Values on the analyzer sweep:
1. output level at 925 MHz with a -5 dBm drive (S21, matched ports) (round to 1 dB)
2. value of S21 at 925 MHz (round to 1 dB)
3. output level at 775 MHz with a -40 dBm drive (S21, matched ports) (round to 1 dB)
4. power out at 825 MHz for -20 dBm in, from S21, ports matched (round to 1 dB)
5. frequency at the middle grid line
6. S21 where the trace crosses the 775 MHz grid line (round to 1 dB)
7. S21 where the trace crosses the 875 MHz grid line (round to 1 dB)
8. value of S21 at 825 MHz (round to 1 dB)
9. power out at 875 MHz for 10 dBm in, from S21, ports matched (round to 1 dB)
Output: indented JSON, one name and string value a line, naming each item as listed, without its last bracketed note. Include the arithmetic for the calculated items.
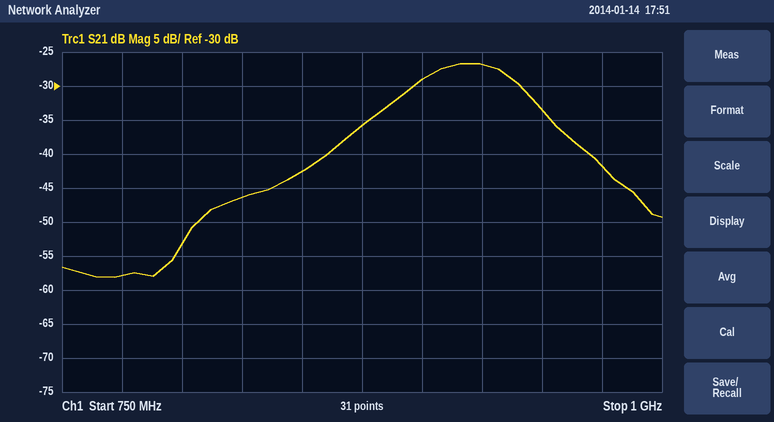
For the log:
{
  "output level at 925 MHz with a -5 dBm drive (S21, matched ports)": "-5 dBm + (-27 dB) = -32 dBm",
  "value of S21 at 925 MHz": "-27 dB",
  "output level at 775 MHz with a -40 dBm drive (S21, matched ports)": "-40 dBm + (-58 dB) = -98 dBm",
  "power out at 825 MHz for -20 dBm in, from S21, ports matched": "-20 dBm + (-46 dB) = -66 dBm",
  "frequency at the middle grid line": "875 MHz",
  "S21 where the trace crosses the 775 MHz grid line": "-58 dB",
  "S21 where the trace crosses the 875 MHz grid line": "-36 dB",
  "value of S21 at 825 MHz": "-46 dB",
  "power out at 875 MHz for 10 dBm in, from S21, ports matched": "10 dBm + (-36 dB) = -26 dBm"
}
